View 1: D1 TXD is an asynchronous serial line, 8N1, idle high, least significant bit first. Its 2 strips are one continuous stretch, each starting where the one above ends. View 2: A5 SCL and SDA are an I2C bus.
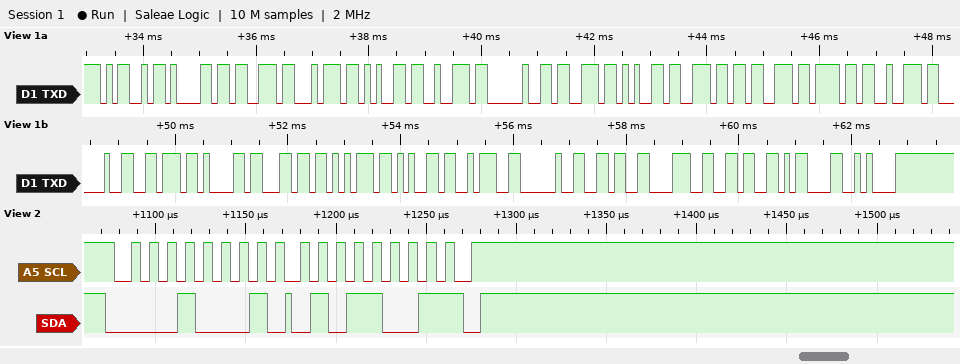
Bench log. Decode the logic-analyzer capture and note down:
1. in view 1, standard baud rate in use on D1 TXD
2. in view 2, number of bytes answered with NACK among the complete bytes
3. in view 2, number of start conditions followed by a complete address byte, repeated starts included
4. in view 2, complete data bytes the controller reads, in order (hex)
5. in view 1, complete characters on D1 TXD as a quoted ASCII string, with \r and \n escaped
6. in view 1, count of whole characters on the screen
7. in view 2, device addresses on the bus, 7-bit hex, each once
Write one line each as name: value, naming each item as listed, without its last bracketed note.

in view 1, standard baud rate in use on D1 TXD: 9600 baud
in view 2, number of bytes answered with NACK among the complete bytes: 1
in view 2, number of start conditions followed by a complete address byte, repeated starts included: 1
in view 2, complete data bytes the controller reads, in order: 59
in view 1, complete characters on D1 TXD as a quoted ASCII string, with \r and \n escaped: "Master sensor value: 686\r\n"
in view 1, count of whole characters on the screen: 26
in view 2, device addresses on the bus, 7-bit hex, each once: 0x08
